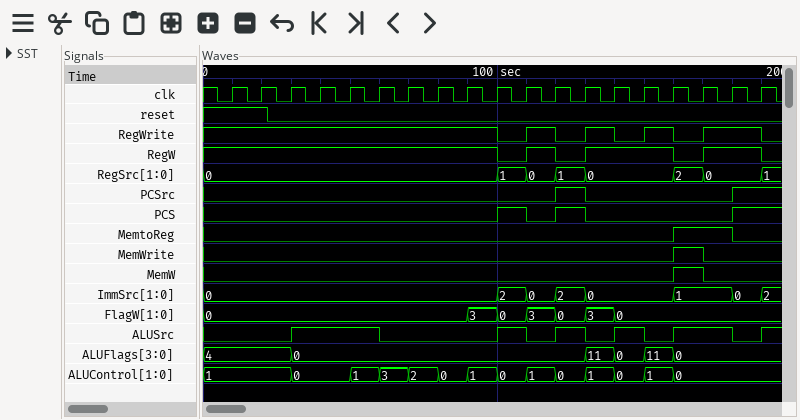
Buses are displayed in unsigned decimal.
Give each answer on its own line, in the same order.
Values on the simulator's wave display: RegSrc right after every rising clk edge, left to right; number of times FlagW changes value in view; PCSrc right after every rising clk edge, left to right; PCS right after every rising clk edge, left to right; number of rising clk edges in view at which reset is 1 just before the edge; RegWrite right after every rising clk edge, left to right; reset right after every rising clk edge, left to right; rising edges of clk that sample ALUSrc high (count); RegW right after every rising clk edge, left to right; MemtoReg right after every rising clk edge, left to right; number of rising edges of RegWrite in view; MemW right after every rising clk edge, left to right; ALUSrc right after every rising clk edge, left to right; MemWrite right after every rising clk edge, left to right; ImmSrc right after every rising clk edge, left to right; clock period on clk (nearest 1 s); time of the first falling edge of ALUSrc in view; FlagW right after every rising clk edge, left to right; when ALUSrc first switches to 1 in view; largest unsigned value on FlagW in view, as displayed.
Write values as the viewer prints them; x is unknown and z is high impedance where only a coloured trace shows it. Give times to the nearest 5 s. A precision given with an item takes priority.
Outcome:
0, 0, 0, 0, 0, 0, 0, 0, 0, 1, 0, 1, 0, 0, 0, 2, 0, 0, 1
6
0 0 0 0 0 0 0 0 0 0 0 1 0 0 0 0 0 1 1
0 0 0 0 0 0 0 0 0 1 0 1 0 0 0 0 0 1 1
2
1 1 1 1 1 1 1 1 1 0 1 0 1 0 1 0 1 1 0
1 1 0 0 0 0 0 0 0 0 0 0 0 0 0 0 0 0 0
8
1 1 1 1 1 1 1 1 1 0 1 0 1 1 1 0 1 1 0
0 0 0 0 0 0 0 0 0 0 0 0 0 0 0 1 1 0 0
4
0 0 0 0 0 0 0 0 0 0 0 0 0 0 0 1 0 0 0
0 0 1 1 1 0 0 0 0 1 0 1 0 1 0 1 1 0 1
0 0 0 0 0 0 0 0 0 0 0 0 0 0 0 1 0 0 0
0, 0, 0, 0, 0, 0, 0, 0, 0, 2, 0, 2, 0, 0, 0, 1, 1, 0, 2
10 s
60 s
0, 0, 0, 0, 0, 0, 0, 0, 3, 0, 3, 0, 3, 0, 0, 0, 0, 0, 0
30 s
3
